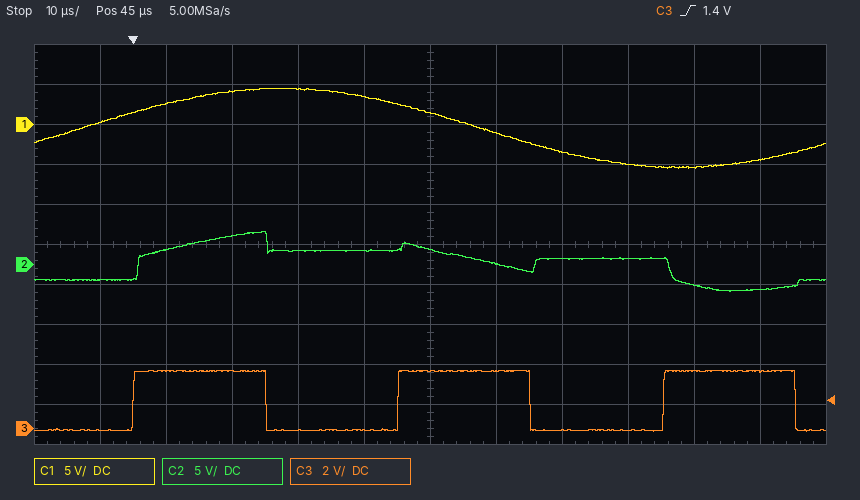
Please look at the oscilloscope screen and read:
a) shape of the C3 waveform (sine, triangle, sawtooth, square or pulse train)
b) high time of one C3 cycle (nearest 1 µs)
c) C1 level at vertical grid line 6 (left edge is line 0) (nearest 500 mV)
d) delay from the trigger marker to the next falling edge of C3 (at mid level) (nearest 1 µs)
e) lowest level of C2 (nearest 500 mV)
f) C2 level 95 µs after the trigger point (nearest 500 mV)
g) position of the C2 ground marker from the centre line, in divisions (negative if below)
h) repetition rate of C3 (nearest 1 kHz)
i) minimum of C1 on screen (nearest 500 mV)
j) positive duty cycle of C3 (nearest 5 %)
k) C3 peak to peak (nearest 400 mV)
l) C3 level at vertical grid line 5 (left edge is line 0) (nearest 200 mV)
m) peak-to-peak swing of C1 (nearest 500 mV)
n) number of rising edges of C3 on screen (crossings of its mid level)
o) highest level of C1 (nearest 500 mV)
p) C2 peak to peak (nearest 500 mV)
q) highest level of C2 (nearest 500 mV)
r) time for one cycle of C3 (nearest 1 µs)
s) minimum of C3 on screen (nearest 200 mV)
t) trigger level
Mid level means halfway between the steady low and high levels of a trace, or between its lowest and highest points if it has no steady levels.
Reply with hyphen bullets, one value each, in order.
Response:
- square
- 20 µs
- 1.5 V
- 20 µs
- -3.5 V
- -3.0 V
- -0.5 div
- 25 kHz
- -5.5 V
- 50 %
- 3.2 V
- 0.0 V
- 10.0 V
- 3
- 4.5 V
- 7.5 V
- 4.0 V
- 40 µs
- -200 mV
- 1.4 V
